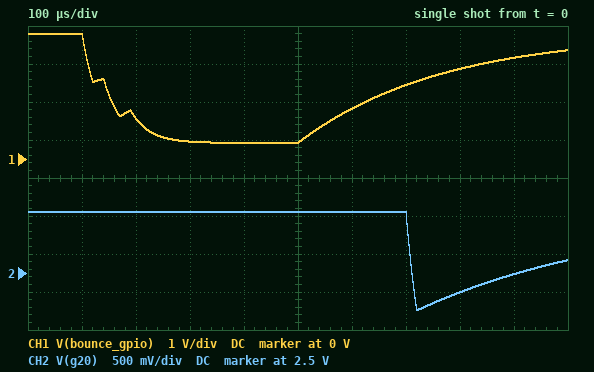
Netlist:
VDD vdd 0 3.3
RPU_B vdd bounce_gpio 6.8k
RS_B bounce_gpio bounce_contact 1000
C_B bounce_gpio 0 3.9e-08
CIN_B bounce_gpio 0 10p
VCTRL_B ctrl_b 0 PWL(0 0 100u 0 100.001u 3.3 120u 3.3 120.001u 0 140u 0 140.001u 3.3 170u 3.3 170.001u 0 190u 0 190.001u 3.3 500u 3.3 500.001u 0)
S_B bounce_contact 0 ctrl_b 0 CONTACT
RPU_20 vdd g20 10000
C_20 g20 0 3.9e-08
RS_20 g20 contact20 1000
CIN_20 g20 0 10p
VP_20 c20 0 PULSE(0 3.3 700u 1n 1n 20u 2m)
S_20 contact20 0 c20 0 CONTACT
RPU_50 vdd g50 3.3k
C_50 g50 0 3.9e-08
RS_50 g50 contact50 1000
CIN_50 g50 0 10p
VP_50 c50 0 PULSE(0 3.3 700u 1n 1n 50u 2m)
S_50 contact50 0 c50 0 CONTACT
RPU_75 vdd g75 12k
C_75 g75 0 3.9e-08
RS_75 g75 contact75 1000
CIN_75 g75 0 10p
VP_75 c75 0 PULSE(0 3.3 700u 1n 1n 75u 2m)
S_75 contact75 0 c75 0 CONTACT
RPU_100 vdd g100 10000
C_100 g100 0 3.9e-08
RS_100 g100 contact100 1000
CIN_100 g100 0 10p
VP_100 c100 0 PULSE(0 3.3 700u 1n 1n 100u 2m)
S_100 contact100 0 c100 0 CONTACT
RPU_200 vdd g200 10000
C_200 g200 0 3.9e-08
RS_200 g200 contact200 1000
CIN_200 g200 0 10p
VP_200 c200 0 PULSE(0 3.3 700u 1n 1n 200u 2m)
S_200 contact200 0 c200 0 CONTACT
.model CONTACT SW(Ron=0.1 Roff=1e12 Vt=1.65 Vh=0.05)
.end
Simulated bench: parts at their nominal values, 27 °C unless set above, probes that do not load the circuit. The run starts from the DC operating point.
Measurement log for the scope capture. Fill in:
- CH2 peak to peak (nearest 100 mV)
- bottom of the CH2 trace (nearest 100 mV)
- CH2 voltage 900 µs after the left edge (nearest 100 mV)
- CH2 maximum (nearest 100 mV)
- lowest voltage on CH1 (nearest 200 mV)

1.3 V
2.0 V
2.5 V
3.3 V
400 mV
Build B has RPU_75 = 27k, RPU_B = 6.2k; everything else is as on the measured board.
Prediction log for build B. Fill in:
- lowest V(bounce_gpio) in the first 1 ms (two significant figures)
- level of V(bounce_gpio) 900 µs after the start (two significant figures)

460 mV
2.8 V
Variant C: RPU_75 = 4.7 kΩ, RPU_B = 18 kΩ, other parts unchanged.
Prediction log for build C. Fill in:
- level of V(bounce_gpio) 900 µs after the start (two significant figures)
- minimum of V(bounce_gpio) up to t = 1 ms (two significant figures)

1.5 V
170 mV
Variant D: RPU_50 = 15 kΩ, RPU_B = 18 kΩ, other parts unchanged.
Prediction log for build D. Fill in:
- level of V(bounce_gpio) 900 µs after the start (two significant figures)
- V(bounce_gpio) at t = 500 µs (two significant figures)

1.5 V
170 mV
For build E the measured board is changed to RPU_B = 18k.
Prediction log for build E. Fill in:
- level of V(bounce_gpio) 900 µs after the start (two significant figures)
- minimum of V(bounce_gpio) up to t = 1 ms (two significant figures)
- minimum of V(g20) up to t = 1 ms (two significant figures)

1.5 V
170 mV
2.0 V
